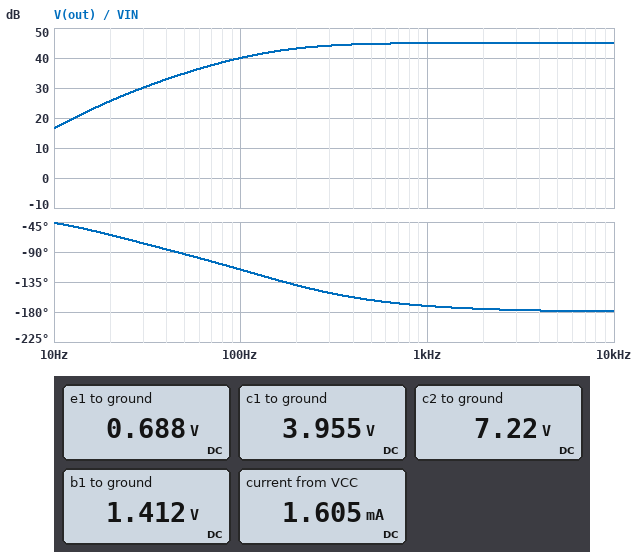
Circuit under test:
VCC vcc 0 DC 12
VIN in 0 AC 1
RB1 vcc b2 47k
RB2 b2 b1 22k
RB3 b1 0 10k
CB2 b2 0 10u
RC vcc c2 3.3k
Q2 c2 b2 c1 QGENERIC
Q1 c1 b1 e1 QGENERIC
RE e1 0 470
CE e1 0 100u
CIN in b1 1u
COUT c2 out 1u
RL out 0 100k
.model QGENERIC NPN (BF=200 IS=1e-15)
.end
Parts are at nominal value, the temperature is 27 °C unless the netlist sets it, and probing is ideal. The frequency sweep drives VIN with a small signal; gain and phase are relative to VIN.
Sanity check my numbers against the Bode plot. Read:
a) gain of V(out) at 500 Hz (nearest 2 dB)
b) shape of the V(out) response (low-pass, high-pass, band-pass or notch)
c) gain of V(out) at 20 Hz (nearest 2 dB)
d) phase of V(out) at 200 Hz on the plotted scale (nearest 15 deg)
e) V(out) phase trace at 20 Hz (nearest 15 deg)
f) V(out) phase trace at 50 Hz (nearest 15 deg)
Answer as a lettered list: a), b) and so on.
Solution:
a) 44 dB
b) high-pass
c) 26 dB
d) -135 deg
e) -60 deg
f) -90 deg
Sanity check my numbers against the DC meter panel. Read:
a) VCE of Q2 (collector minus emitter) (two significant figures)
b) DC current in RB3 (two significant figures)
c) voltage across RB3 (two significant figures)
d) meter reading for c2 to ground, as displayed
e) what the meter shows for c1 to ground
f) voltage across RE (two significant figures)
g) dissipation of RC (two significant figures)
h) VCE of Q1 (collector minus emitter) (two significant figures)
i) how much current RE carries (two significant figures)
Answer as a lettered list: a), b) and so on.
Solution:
a) 3.3 V
b) 140 µA
c) 1.4 V
d) 7.22 V
e) 3.955 V
f) 690 mV
g) 6.9 mW
h) 3.3 V
i) 1.5 mA
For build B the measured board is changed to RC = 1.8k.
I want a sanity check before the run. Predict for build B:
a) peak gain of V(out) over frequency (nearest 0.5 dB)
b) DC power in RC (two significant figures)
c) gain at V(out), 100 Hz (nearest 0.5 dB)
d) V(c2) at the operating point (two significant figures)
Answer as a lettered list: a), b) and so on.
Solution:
a) 40.0 dB
b) 3.8 mW
c) 35.0 dB
d) 9.4 V
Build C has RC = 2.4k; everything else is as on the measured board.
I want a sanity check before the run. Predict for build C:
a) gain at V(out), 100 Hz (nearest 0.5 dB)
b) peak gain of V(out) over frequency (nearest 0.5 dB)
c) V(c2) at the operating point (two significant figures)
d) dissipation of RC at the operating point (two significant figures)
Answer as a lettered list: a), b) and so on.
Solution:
a) 37.5 dB
b) 42.5 dB
c) 8.5 V
d) 5.0 mW
